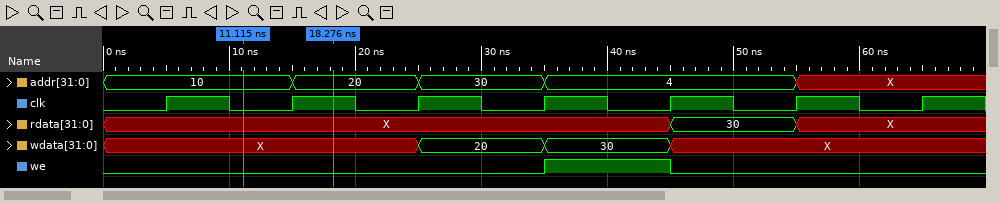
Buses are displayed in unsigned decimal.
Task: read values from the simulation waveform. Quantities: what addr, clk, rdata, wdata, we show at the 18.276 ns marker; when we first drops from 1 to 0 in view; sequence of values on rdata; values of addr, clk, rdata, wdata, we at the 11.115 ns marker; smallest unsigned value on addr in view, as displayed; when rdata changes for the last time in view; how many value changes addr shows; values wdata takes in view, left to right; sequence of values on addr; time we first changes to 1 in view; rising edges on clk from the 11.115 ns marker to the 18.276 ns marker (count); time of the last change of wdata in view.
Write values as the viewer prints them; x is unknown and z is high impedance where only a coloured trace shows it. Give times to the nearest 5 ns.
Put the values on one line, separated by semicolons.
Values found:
addr=20, clk=1, rdata=X, wdata=X, we=0; 45 ns; X, 30, X; addr=10, clk=0, rdata=X, wdata=X, we=0; 4; 55 ns; 4; X, 20, 30, X; 10, 20, 30, 4, X; 35 ns; 1; 45 ns
